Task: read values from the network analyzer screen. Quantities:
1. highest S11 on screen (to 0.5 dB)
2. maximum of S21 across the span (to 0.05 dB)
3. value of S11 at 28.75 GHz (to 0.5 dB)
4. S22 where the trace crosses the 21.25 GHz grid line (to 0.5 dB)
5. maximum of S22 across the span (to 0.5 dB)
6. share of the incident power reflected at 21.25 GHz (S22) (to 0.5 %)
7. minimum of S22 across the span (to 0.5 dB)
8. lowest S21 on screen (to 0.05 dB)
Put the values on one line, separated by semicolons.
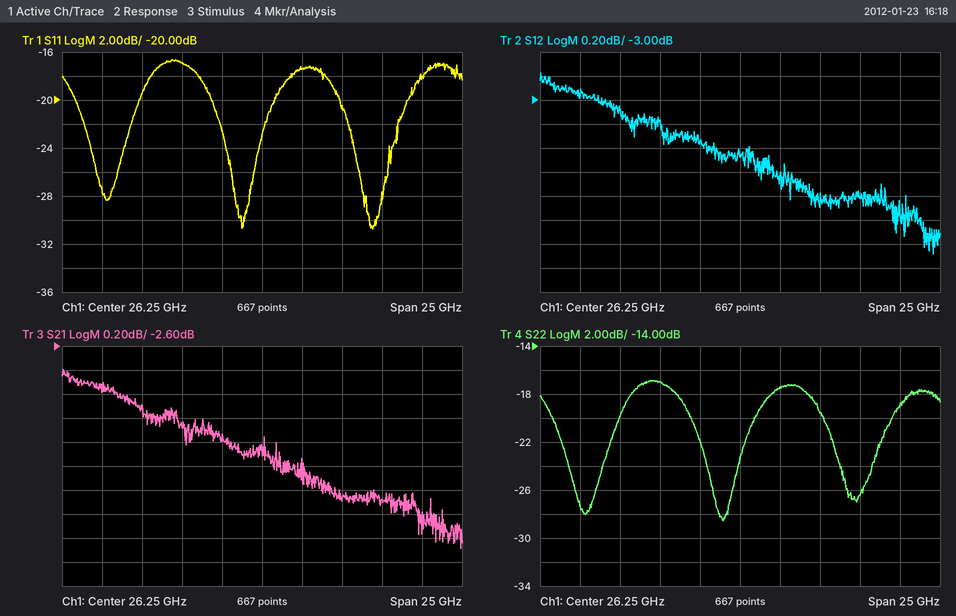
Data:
-16.5 dB; -2.80 dB; -17.5 dB; -17.0 dB; -17.0 dB; 2.0 %; -28.5 dB; -4.30 dB
